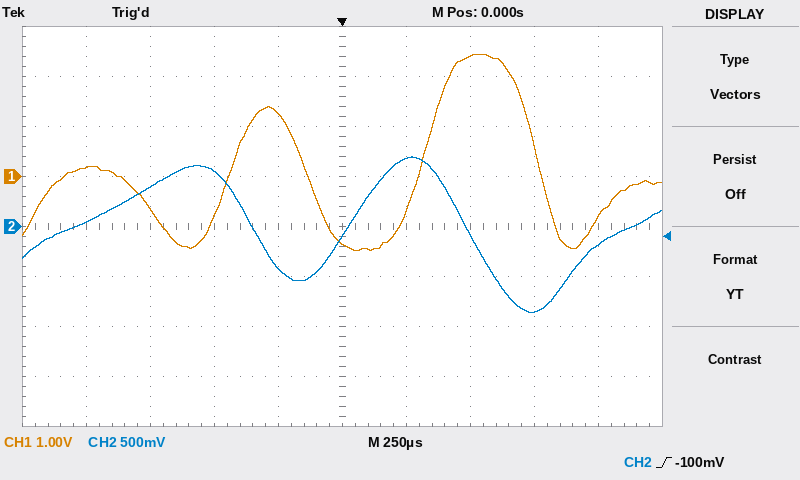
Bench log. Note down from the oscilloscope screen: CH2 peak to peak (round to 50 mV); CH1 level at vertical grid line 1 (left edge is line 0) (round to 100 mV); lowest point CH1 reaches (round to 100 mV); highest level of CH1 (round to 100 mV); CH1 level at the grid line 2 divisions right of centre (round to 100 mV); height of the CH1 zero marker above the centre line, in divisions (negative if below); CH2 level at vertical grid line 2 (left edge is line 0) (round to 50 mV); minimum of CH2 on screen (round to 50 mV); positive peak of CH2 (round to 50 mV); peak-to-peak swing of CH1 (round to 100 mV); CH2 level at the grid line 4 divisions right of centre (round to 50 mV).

1.55 V
200 mV
-1.5 V
2.4 V
2.4 V
+1.0 div
400 mV
-850 mV
700 mV
3.9 V
-200 mV
